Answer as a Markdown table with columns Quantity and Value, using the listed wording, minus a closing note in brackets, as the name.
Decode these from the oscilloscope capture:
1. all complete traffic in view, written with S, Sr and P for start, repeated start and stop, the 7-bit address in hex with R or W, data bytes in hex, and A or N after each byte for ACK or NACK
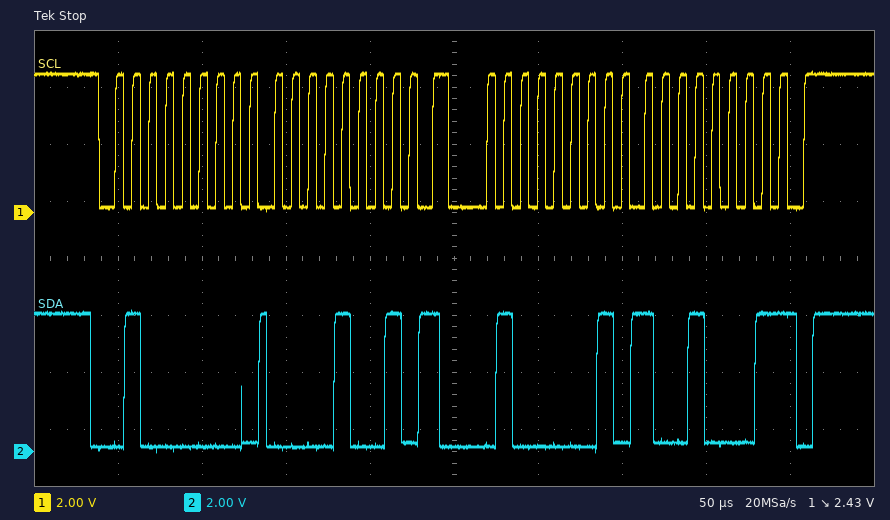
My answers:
| Quantity | Value |
|---|---|
| all complete traffic in view, written with S, Sr and P for start, repeated start and stop, the 7-bit address in hex with R or W, data bytes in hex, and A or N after each byte for ACK or NACK | S 20W A 09 A Sr 20R A 91 N P |
